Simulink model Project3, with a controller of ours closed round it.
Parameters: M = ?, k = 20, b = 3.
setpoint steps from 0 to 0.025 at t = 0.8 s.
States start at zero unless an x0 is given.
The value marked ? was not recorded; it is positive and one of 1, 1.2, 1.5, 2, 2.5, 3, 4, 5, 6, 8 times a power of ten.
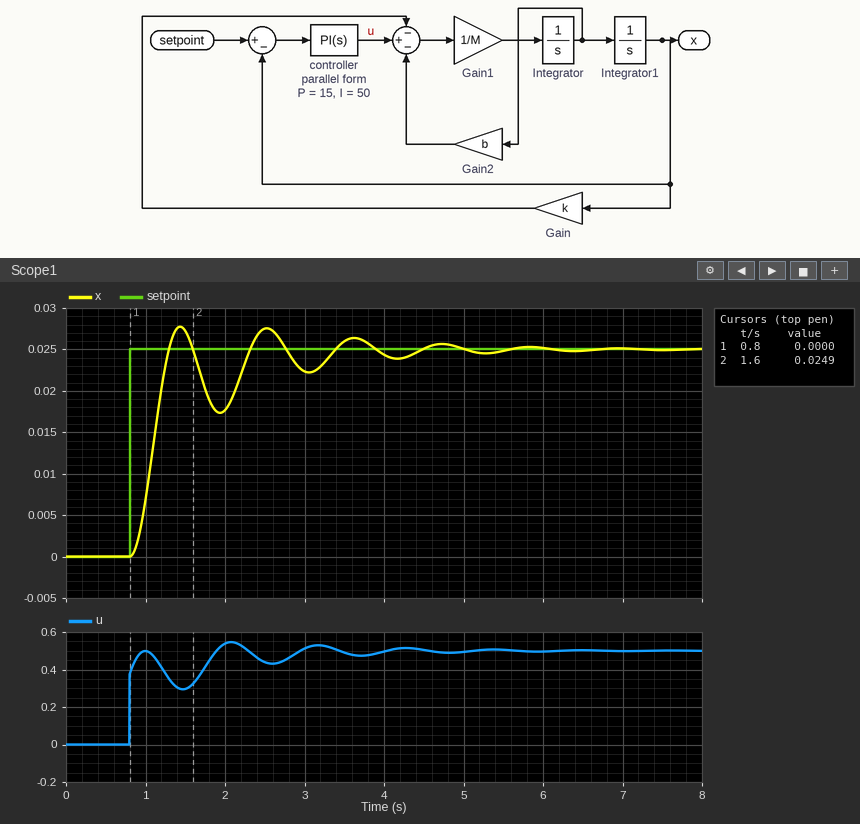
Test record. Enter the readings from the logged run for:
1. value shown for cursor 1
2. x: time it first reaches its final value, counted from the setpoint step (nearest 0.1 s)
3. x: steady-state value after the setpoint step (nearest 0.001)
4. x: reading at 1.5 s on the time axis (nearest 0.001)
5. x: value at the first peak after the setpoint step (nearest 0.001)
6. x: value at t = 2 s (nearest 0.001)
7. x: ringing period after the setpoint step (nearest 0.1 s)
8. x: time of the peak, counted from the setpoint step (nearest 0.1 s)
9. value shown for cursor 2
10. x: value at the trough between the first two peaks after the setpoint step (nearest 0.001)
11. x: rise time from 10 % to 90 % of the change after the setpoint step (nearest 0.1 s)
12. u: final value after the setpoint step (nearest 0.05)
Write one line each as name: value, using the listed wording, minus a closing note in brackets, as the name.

value shown for cursor 1: 0.0000
x: time it first reaches its final value, counted from the setpoint step: 0.5 s
x: steady-state value after the setpoint step: 0.025
x: reading at 1.5 s on the time axis: 0.027
x: value at the first peak after the setpoint step: 0.028
x: value at t = 2 s: 0.018
x: ringing period after the setpoint step: 1.1 s
x: time of the peak, counted from the setpoint step: 0.6 s
value shown for cursor 2: 0.0249
x: value at the trough between the first two peaks after the setpoint step: 0.017
x: rise time from 10 % to 90 % of the change after the setpoint step: 0.3 s
u: final value after the setpoint step: 0.50
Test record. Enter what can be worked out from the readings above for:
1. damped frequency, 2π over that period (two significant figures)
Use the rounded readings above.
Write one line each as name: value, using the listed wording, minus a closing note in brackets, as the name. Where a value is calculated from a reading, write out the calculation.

damped frequency, 2π over that period: 2π / 1.1 = 5.7 rad/s
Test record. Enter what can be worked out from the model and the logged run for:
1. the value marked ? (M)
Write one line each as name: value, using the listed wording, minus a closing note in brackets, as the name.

the value marked ?: 1
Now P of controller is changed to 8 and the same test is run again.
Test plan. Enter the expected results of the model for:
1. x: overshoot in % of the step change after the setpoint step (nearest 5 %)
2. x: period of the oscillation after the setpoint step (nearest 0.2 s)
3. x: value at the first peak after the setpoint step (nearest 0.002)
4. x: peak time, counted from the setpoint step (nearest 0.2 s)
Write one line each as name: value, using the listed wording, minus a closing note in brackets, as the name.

x: overshoot in % of the step change after the setpoint step: 15 %
x: period of the oscillation after the setpoint step: 1.2 s
x: value at the first peak after the setpoint step: 0.028
x: peak time, counted from the setpoint step: 0.8 s
